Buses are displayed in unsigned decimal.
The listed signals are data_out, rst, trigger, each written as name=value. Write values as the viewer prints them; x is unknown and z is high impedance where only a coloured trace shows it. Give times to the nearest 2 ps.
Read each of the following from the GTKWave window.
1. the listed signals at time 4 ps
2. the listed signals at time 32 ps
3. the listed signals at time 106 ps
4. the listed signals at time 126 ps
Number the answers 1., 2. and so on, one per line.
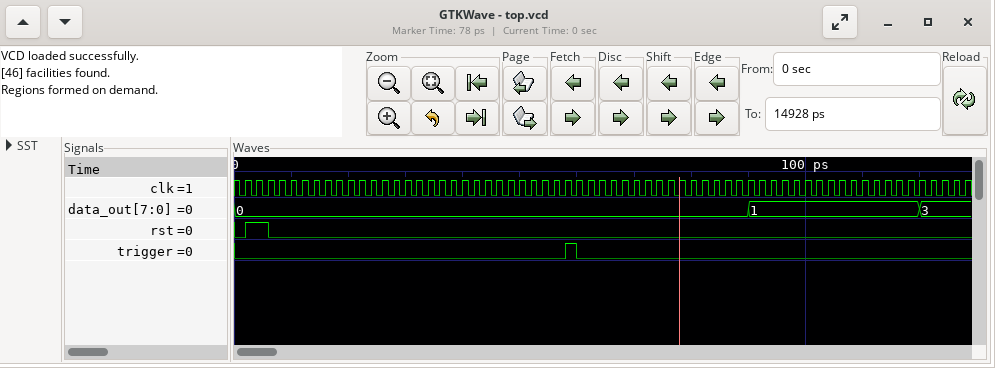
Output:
1. data_out=0, rst=1, trigger=0
2. data_out=0, rst=0, trigger=0
3. data_out=1, rst=0, trigger=0
4. data_out=3, rst=0, trigger=0
